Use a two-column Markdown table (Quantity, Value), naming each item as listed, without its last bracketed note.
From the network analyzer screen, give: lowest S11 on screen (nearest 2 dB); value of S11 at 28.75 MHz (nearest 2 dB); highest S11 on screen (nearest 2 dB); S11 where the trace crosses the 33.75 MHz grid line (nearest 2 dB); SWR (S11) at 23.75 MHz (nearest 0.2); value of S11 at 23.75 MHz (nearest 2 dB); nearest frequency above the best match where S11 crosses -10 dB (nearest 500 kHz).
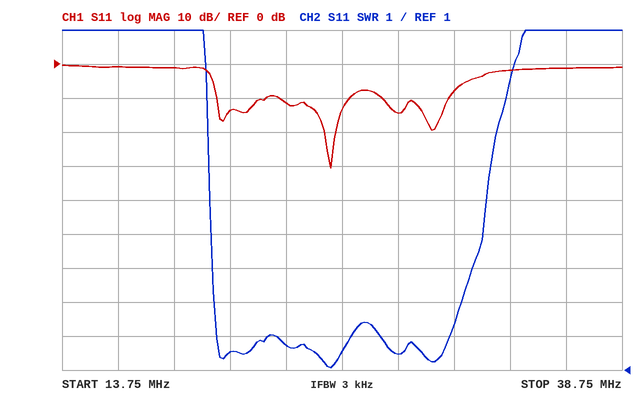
| Quantity | Value |
|---|---|
| lowest S11 on screen | -30 dB |
| value of S11 at 28.75 MHz | -14 dB |
| highest S11 on screen | 0 dB |
| S11 where the trace crosses the 33.75 MHz grid line | -2 dB |
| SWR (S11) at 23.75 MHz | 1.8 |
| value of S11 at 23.75 MHz | -12 dB |
| nearest frequency above the best match where S11 crosses -10 dB | 26.5 MHz |
